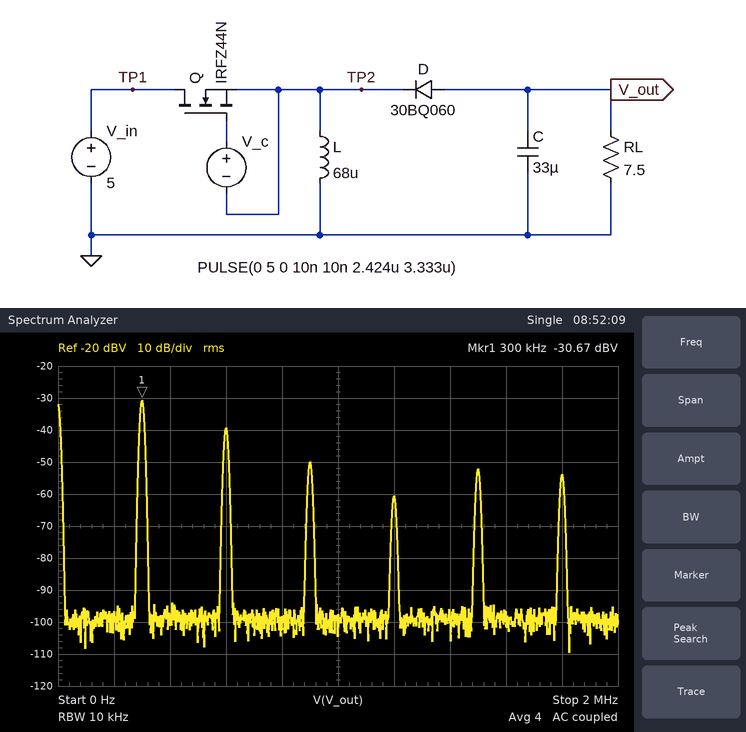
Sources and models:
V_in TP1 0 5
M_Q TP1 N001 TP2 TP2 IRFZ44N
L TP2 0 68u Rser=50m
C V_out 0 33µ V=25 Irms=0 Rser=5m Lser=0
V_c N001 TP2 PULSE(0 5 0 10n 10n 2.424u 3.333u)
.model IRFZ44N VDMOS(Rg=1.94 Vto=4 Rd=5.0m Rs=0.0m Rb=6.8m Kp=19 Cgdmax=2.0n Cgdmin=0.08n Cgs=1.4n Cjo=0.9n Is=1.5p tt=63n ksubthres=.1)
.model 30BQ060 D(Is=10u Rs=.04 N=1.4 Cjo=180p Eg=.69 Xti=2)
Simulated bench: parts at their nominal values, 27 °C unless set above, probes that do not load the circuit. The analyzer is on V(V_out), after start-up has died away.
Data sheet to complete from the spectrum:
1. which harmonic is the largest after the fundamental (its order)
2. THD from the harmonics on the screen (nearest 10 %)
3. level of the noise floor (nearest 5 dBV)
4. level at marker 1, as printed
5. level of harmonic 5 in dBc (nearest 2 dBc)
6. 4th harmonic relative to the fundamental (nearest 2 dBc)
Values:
2
40 %
-100 dBV
-30.67 dBV
-22 dBc
-30 dBc
